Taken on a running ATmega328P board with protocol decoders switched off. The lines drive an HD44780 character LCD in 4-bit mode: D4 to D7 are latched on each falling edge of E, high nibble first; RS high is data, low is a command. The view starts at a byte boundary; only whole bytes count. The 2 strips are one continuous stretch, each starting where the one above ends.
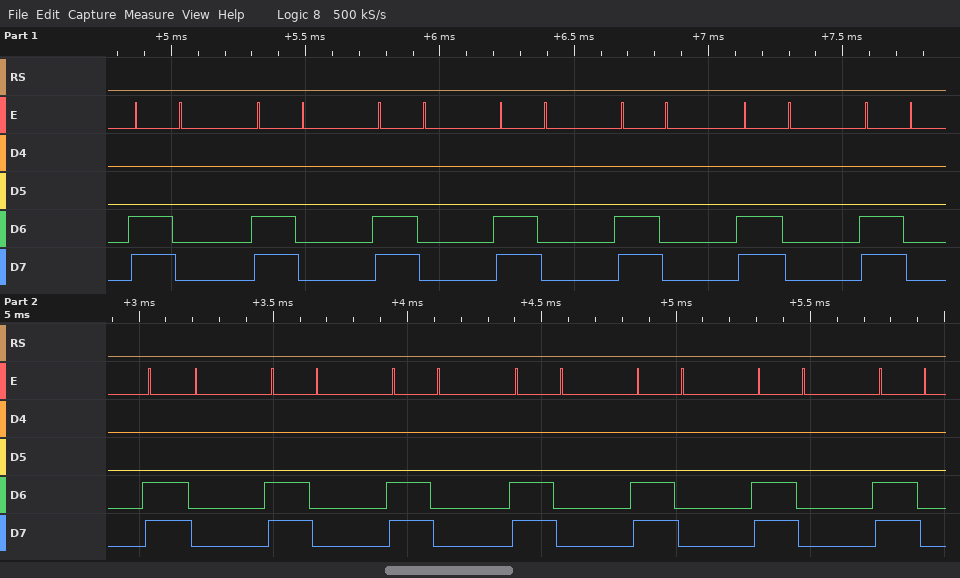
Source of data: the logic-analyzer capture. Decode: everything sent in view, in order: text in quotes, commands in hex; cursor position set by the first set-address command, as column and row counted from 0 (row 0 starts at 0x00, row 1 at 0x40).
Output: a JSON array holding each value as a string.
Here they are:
["0xC0 0xC0 0xC0 0xC0 0xC0 0xC0 0xC0 0xC0 0xC0 0xC0 0xC0 0xC0 0xC0 0xC0", "column 0, row 1"]
